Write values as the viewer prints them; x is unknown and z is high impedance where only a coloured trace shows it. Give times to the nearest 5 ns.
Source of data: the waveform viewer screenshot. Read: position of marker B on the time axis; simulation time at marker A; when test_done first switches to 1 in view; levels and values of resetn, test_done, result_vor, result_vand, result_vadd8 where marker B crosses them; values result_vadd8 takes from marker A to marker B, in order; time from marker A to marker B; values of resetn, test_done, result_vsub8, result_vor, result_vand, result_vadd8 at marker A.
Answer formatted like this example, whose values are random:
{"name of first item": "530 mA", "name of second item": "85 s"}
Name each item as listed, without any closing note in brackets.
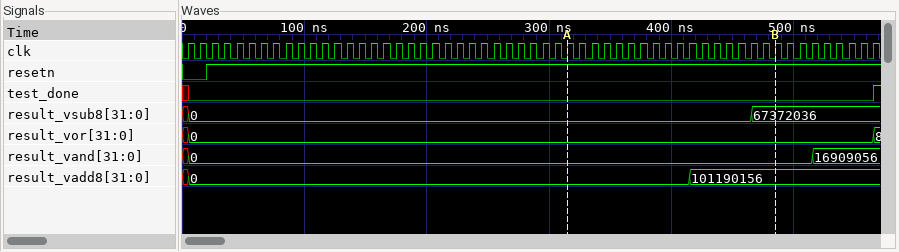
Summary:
{"position of marker B on the time axis": "485 ns", "simulation time at marker A": "315 ns", "when test_done first switches to 1 in view": "565 ns", "levels and values of resetn, test_done, result_vor, result_vand, result_vadd8 where marker B crosses them": "resetn=1, test_done=0, result_vor=0, result_vand=0, result_vadd8=101190156", "values result_vadd8 takes from marker A to marker B, in order": "0, 101190156", "time from marker A to marker B": "170 ns", "values of resetn, test_done, result_vsub8, result_vor, result_vand, result_vadd8 at marker A": "resetn=1, test_done=0, result_vsub8=0, result_vor=0, result_vand=0, result_vadd8=0"}
